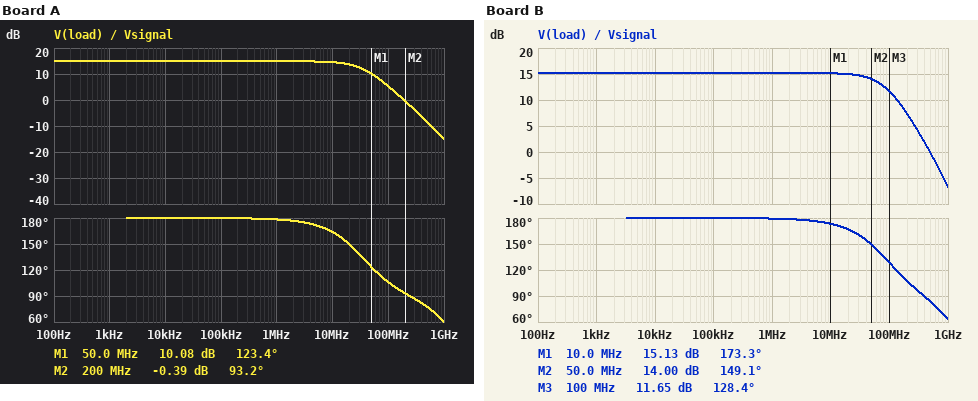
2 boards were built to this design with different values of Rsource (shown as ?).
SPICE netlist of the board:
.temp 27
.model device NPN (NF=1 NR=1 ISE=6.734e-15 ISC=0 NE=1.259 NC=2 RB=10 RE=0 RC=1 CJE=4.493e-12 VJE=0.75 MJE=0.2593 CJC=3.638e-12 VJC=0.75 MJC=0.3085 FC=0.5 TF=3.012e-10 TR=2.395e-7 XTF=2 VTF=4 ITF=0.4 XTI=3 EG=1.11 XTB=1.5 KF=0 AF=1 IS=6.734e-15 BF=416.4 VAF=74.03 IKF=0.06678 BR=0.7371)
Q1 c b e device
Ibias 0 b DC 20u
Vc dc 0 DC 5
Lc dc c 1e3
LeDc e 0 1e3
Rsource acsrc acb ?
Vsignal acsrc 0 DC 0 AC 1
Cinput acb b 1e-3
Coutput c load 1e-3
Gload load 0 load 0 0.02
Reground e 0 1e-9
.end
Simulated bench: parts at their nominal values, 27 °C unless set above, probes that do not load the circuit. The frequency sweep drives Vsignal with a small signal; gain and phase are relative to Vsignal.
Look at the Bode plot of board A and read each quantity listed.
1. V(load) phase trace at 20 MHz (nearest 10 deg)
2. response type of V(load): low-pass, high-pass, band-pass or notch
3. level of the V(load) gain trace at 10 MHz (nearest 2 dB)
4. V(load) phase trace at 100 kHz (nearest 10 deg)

150 deg
low-pass
14 dB
180 deg
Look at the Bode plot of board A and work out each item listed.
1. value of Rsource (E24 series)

75 Ω
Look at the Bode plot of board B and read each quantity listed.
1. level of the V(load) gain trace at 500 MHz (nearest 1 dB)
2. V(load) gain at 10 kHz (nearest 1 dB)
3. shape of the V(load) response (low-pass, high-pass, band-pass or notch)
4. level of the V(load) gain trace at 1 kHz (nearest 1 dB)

0 dB
15 dB
low-pass
15 dB
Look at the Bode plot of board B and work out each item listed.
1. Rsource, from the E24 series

22 Ω
